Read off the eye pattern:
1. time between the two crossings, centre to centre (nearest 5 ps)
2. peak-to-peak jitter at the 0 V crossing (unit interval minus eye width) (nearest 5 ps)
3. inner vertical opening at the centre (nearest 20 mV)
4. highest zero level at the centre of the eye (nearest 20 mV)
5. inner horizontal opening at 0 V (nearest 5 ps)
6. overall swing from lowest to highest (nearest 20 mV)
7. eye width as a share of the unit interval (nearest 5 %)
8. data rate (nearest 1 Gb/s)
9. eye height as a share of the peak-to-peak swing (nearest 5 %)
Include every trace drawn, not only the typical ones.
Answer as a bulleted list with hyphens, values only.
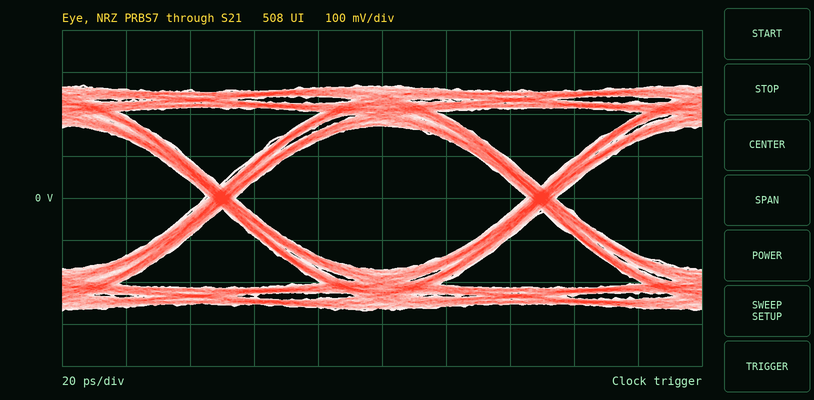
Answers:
- 100 ps
- 10 ps
- 340 mV
- -180 mV
- 90 ps
- 540 mV
- 90 %
- 10 Gb/s
- 65 %
